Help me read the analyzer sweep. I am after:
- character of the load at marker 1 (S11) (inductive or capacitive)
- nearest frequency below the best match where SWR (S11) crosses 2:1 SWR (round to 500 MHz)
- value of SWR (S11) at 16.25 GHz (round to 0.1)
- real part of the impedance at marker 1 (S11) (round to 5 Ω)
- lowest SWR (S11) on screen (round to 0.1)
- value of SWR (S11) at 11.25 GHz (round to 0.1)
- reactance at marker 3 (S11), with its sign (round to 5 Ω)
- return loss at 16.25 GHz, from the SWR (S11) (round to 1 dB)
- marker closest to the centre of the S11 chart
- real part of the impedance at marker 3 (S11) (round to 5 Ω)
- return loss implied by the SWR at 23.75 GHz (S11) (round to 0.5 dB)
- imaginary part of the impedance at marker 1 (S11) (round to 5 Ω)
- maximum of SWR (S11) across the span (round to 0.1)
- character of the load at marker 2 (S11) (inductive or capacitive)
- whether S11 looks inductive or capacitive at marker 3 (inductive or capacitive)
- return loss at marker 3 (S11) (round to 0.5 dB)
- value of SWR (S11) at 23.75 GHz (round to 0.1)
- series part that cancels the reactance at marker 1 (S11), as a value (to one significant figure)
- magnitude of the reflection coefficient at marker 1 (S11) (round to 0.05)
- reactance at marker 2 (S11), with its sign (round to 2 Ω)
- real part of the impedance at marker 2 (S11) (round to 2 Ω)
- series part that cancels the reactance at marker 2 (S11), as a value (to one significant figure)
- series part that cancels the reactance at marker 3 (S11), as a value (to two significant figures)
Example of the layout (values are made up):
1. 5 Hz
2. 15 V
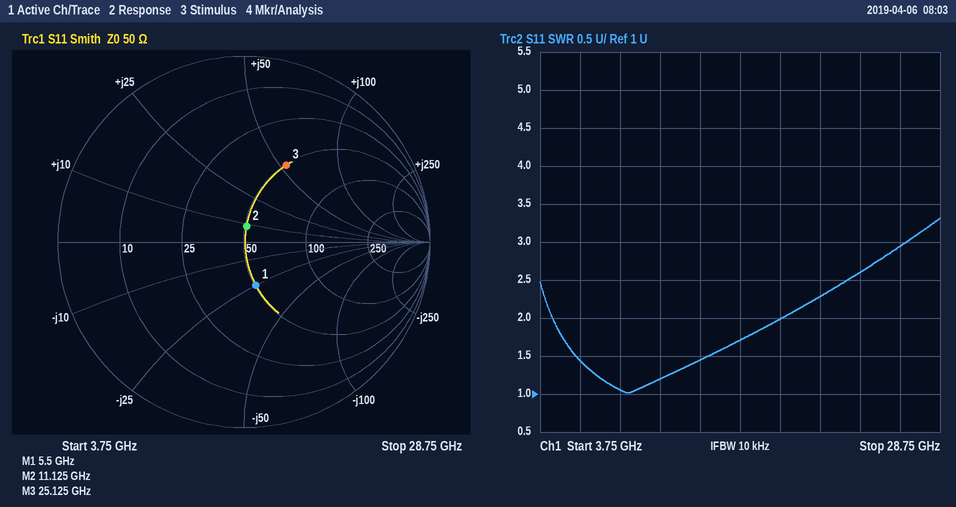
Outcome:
1. capacitive
2. 4.5 GHz
3. 1.7
4. 50 Ω
5. 1.0
6. 1.2
7. +55 Ω
8. 12 dB
9. marker 2
10. 50 Ω
11. 7.0 dB
12. -25 Ω
13. 3.3
14. inductive
15. inductive
16. 6.5 dB
17. 2.6
18. 700 pH
19. 0.25
20. +8 Ω
21. 50 Ω
22. 2 pF
23. 120 fF
